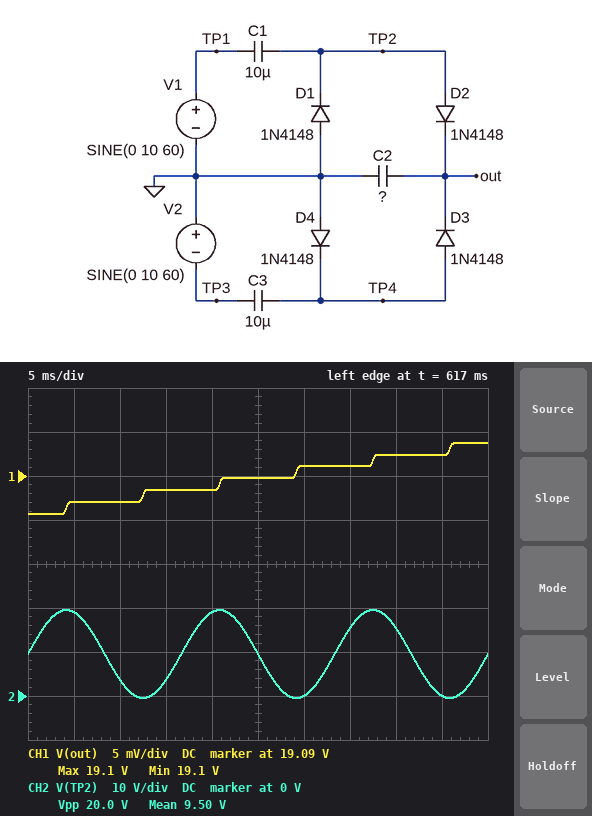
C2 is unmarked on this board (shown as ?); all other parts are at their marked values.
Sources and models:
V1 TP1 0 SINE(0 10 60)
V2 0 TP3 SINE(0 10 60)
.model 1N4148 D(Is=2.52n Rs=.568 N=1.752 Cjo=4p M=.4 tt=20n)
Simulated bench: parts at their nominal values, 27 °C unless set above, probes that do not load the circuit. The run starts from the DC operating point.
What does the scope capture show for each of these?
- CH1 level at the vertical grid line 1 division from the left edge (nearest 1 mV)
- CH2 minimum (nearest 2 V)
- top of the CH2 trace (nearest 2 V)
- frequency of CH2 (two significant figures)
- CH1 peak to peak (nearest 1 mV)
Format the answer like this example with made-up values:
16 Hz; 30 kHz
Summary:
19.087 V; 0 V; 20 V; 60 Hz; 8 mV
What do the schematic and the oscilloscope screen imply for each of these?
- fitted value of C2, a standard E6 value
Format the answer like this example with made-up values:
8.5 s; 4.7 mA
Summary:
15 µF
